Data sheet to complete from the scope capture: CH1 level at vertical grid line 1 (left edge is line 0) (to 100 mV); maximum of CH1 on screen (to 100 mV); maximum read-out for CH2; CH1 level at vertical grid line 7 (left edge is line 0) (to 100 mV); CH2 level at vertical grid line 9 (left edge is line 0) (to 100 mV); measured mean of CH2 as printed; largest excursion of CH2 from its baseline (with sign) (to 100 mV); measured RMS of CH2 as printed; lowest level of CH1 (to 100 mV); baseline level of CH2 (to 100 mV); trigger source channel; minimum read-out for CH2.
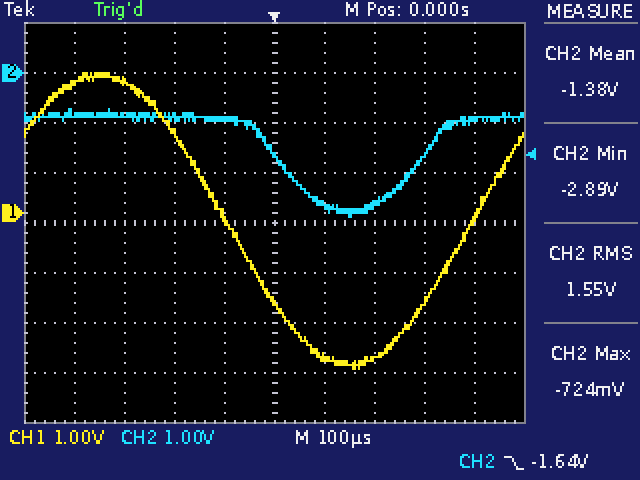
2.6 V
2.8 V
-724 mV
-2.9 V
-900 mV
-1.38 V
-2.0 V
1.55 V
-3.1 V
-900 mV
CH2
-2.89 V
